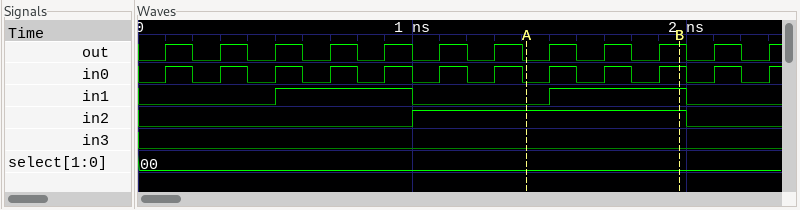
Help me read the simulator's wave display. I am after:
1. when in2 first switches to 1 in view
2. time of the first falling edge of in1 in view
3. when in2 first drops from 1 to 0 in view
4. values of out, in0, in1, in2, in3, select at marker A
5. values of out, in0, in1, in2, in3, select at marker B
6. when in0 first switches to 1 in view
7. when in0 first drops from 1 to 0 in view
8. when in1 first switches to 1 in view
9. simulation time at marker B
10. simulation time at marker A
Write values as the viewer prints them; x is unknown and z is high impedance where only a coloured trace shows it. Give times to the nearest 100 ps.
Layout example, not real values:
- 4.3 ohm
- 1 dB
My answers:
- 1000 ps
- 1000 ps
- 2000 ps
- out=0, in0=0, in1=0, in2=1, in3=0, select=00
- out=1, in0=1, in1=1, in2=1, in3=0, select=00
- 100 ps
- 200 ps
- 500 ps
- 2000 ps
- 1400 ps
